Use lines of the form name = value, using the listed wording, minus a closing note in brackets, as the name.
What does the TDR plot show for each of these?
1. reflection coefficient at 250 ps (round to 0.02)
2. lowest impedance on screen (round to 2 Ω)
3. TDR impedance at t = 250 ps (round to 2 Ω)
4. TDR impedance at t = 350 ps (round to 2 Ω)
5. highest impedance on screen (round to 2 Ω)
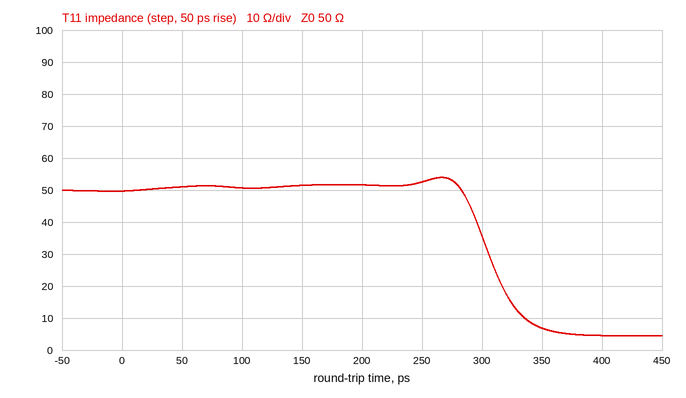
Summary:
reflection coefficient at 250 ps = +0.02
lowest impedance on screen = 4 Ω
TDR impedance at t = 250 ps = 52 Ω
TDR impedance at t = 350 ps = 6 Ω
highest impedance on screen = 54 Ω
